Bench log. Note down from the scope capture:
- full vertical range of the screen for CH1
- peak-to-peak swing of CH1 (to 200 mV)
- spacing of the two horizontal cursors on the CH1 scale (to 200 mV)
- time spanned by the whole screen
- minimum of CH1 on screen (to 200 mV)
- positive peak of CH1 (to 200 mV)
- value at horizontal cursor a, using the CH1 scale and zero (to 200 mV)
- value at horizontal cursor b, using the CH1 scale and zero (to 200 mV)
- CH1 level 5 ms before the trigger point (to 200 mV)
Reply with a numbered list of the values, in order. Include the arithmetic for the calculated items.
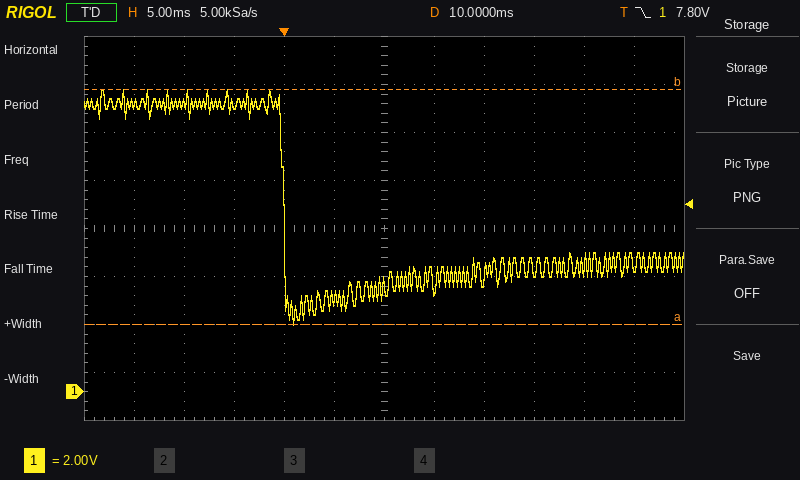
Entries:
1. 16 V
2. 12.6 V − (2.8 V) = 9.8 V
3. 9.8 V
4. 60 ms
5. 2.8 V
6. 12.6 V
7. 2.8 V
8. 12.6 V
9. 12.0 V
